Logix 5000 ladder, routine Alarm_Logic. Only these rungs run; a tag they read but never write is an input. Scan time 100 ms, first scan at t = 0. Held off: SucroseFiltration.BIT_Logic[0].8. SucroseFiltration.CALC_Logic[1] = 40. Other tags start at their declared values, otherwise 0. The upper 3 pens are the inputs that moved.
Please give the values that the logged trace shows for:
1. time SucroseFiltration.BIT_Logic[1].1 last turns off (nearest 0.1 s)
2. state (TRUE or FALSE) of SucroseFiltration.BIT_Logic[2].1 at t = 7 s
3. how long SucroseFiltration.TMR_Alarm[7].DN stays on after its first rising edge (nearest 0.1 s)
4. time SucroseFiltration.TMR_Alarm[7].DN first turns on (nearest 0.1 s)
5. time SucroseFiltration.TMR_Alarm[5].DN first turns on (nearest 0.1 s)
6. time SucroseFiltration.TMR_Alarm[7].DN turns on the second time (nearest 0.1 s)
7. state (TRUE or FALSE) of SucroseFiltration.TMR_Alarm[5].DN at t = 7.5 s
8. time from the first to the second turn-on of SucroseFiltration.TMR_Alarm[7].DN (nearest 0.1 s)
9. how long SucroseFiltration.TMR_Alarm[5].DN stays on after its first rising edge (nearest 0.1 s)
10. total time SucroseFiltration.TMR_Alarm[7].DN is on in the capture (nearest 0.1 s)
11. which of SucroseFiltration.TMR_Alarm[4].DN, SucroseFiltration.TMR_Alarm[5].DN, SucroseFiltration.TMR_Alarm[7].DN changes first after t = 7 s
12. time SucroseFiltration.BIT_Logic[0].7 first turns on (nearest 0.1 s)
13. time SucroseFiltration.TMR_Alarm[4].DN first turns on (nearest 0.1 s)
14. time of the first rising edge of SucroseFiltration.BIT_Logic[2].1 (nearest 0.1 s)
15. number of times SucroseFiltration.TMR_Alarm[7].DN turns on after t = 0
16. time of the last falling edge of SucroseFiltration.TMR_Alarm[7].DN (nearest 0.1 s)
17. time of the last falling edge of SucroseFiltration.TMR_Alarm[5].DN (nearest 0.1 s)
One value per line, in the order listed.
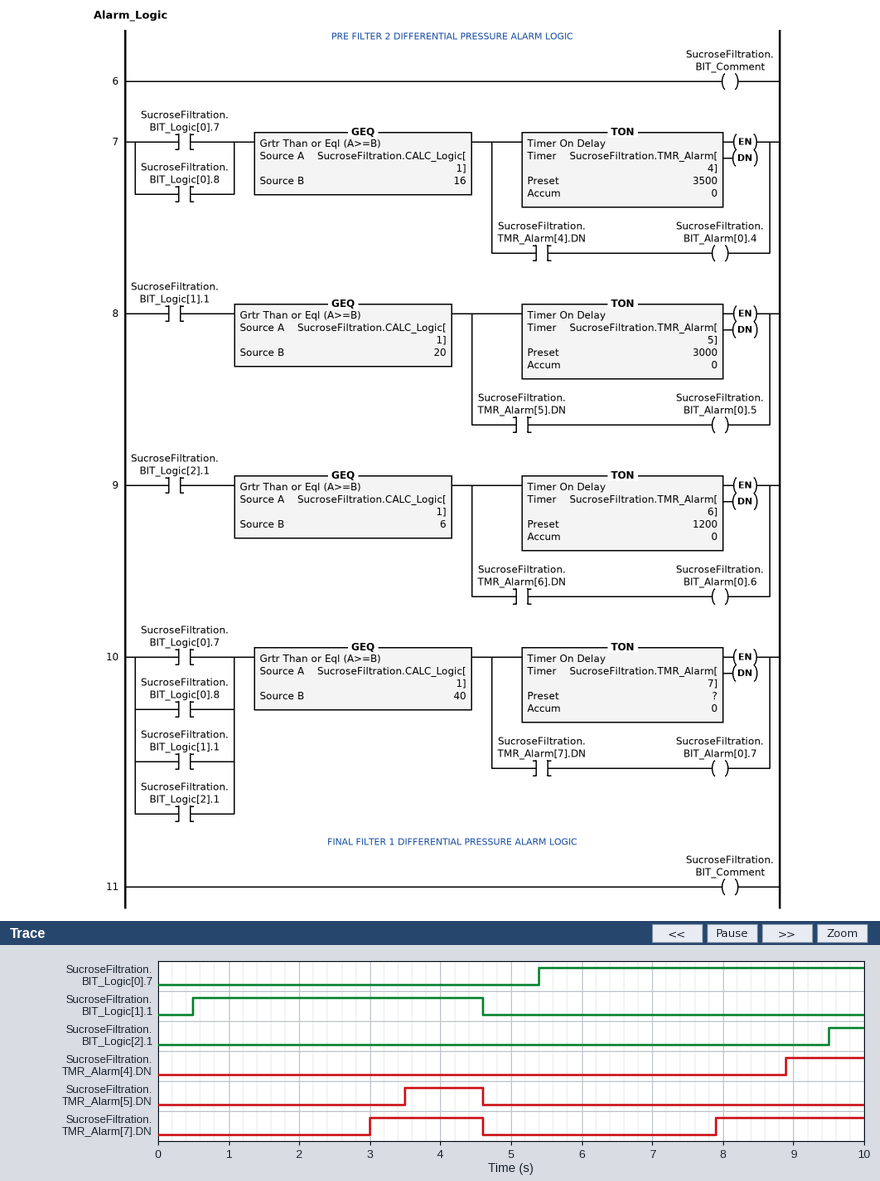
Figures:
4.6 s
FALSE
1.6 s
3.0 s
3.5 s
7.9 s
FALSE
4.9 s
1.1 s
3.7 s
SucroseFiltration.TMR_Alarm[7].DN
5.4 s
8.9 s
9.5 s
2
4.6 s
4.6 s
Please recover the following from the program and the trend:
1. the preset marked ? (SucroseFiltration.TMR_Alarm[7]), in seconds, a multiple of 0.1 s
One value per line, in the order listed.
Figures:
2.5 s
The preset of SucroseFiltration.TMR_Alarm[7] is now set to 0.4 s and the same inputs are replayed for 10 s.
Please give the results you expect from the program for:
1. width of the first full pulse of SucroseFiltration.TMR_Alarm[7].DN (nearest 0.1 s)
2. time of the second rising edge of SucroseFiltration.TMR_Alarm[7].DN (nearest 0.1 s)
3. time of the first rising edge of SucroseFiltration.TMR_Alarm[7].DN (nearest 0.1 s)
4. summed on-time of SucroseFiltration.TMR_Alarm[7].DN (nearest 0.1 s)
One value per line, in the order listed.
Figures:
3.7 s
5.8 s
0.9 s
7.9 s
